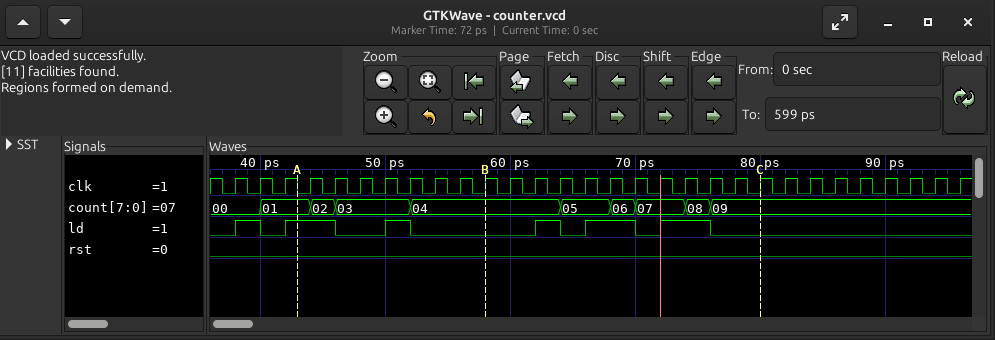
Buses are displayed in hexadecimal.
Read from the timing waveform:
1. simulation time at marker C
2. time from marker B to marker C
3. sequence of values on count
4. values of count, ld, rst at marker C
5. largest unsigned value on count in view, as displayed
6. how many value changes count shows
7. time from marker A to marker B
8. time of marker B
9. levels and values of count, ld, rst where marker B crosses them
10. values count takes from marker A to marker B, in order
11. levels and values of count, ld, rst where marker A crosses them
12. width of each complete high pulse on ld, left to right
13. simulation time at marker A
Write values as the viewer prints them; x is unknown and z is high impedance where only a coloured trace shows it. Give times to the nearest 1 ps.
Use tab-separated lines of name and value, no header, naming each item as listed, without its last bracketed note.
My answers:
simulation time at marker C	80 ps
time from marker B to marker C	22 ps
sequence of values on count	00, 01, 02, 03, 04, 05, 06, 07, 08, 09
values of count, ld, rst at marker C	count=09, ld=0, rst=0
largest unsigned value on count in view, as displayed	09
how many value changes count shows	9
time from marker A to marker B	15 ps
time of marker B	58 ps
levels and values of count, ld, rst where marker B crosses them	count=04, ld=0, rst=0
values count takes from marker A to marker B, in order	01, 02, 03, 04
levels and values of count, ld, rst where marker A crosses them	count=01, ld=1, rst=0
width of each complete high pulse on ld, left to right	2 ps, 4 ps, 2 ps, 2 ps, 4 ps, 4 ps
simulation time at marker A	43 ps
